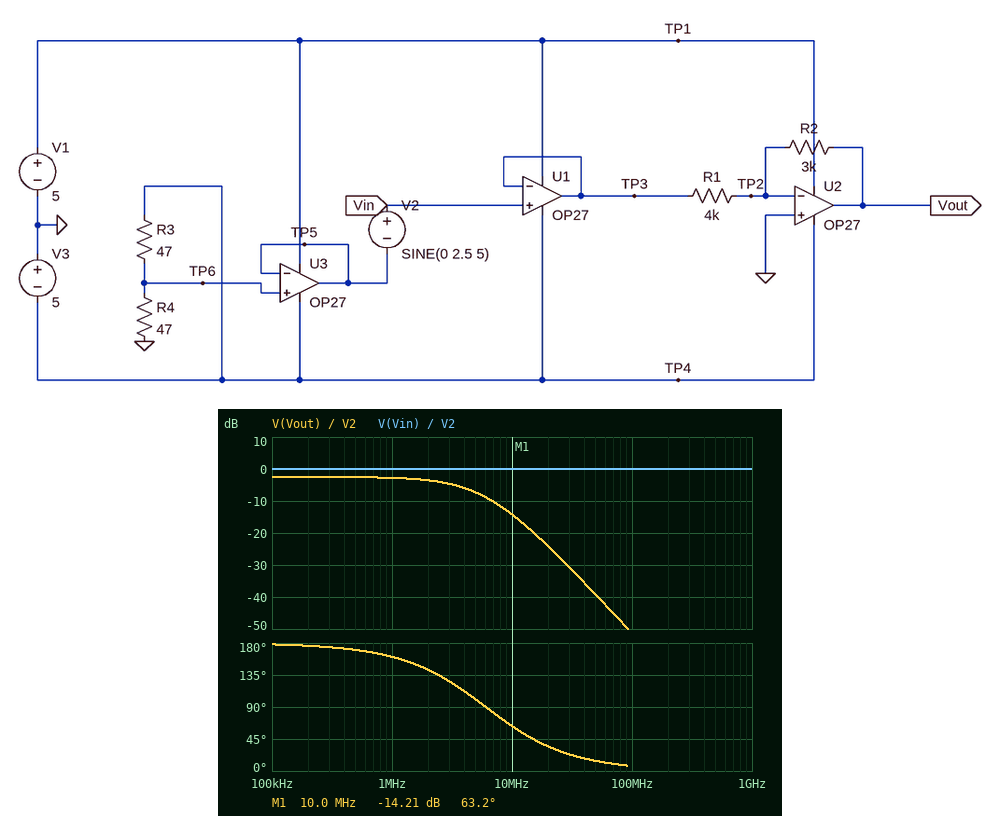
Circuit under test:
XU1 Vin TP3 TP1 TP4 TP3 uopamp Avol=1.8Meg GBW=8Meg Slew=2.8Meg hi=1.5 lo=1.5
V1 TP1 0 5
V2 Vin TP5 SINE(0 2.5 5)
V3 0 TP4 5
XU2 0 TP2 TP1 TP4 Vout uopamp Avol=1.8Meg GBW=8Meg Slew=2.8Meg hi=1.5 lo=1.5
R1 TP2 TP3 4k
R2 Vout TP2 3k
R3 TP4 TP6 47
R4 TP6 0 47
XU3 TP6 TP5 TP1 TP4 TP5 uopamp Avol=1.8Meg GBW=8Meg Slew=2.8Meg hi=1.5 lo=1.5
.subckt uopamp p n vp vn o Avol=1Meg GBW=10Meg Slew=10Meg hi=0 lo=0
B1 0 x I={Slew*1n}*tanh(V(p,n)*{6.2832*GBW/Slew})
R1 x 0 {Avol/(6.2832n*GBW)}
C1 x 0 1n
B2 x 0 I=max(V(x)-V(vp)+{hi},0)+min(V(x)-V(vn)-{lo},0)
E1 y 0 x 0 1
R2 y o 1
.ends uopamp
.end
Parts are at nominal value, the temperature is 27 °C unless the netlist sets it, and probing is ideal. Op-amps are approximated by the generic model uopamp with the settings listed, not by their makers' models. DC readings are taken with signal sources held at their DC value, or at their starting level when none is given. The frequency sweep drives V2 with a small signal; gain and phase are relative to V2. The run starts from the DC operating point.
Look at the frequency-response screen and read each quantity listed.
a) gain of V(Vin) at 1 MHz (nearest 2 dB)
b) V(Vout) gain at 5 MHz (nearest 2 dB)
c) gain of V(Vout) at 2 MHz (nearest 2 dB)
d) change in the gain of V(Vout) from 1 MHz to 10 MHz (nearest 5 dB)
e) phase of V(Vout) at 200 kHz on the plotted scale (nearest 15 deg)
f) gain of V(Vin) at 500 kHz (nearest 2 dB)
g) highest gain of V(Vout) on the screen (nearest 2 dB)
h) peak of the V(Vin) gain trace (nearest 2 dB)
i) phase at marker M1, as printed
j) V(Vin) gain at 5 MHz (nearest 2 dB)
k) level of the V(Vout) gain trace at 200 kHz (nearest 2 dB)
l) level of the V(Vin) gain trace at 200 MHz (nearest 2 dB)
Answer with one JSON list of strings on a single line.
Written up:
["0 dB", "-8 dB", "-4 dB", "-10 dB", "180 deg", "0 dB", "-2 dB", "0 dB", "63.2 deg", "0 dB", "-2 dB", "0 dB"]
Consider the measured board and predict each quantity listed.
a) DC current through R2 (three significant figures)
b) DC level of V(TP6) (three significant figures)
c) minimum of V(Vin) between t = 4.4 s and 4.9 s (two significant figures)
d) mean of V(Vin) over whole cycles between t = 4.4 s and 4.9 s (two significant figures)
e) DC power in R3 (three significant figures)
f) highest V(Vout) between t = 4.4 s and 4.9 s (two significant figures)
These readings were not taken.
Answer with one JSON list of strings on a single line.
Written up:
["625 µA", "-2.50 V", "-5.0 V", "-2.5 V", "133 mW", "2.6 V"]
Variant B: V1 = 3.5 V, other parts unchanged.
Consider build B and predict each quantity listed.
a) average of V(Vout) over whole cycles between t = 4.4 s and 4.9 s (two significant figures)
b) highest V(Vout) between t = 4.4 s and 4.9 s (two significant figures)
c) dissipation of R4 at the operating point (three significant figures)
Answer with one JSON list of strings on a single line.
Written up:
["1.3 V", "2.0 V", "133 mW"]
